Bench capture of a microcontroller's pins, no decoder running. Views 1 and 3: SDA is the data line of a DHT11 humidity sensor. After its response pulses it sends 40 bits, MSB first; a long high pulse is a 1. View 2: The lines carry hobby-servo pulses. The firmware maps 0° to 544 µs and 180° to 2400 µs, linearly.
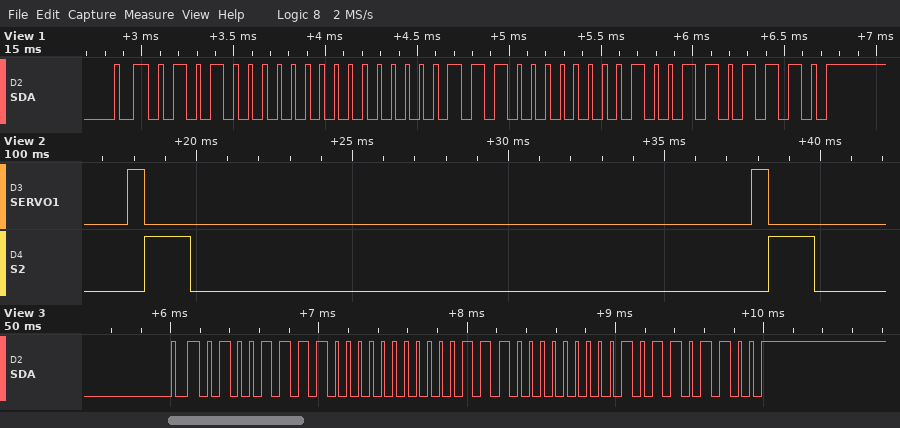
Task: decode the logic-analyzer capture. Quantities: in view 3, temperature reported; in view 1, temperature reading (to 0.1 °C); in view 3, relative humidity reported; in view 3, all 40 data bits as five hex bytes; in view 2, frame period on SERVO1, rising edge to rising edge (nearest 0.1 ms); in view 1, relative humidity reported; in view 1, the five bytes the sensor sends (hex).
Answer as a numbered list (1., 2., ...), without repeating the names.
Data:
1. 28.1 °C
2. 28.2 °C
3. 79 %
4. 4F 00 1C 01 6C
5. 20.0 ms
6. 80 %
7. 50 00 1C 02 6E
